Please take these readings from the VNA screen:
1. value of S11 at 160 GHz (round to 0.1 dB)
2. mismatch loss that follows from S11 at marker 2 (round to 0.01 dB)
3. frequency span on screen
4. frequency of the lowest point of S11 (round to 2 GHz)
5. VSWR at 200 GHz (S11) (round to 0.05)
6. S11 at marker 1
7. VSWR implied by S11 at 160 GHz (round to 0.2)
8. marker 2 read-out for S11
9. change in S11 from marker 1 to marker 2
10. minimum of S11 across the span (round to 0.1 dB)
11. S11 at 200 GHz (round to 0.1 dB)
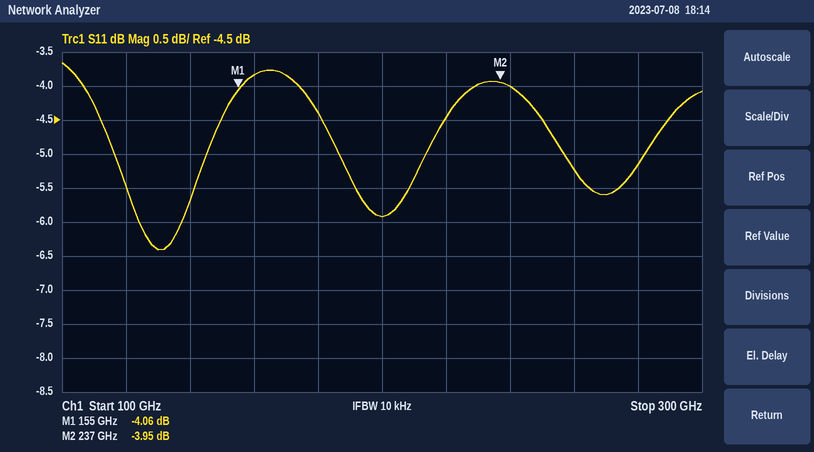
-3.8 dB
2.24 dB
200 GHz
130 GHz
3.05
-4.06 dB
4.6
-3.95 dB
0.11 dB
-6.4 dB
-5.9 dB
